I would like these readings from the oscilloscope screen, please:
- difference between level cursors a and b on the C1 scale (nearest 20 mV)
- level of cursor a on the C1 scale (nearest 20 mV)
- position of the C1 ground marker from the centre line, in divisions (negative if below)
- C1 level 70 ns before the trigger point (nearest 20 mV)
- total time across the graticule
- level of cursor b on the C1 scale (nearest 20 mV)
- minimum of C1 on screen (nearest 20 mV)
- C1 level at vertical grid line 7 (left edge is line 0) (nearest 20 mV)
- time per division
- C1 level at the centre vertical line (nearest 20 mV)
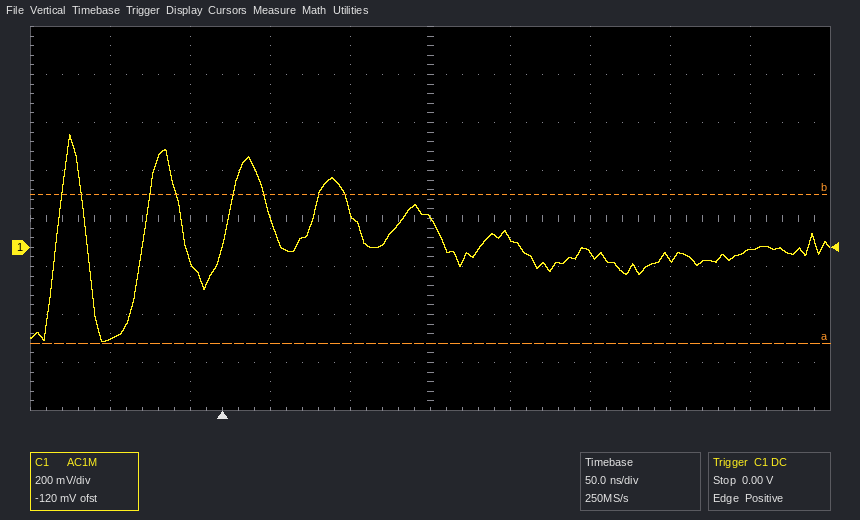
620 mV
-400 mV
-0.6 div
-380 mV
500 ns
220 mV
-400 mV
-20 mV
50 ns
120 mV
